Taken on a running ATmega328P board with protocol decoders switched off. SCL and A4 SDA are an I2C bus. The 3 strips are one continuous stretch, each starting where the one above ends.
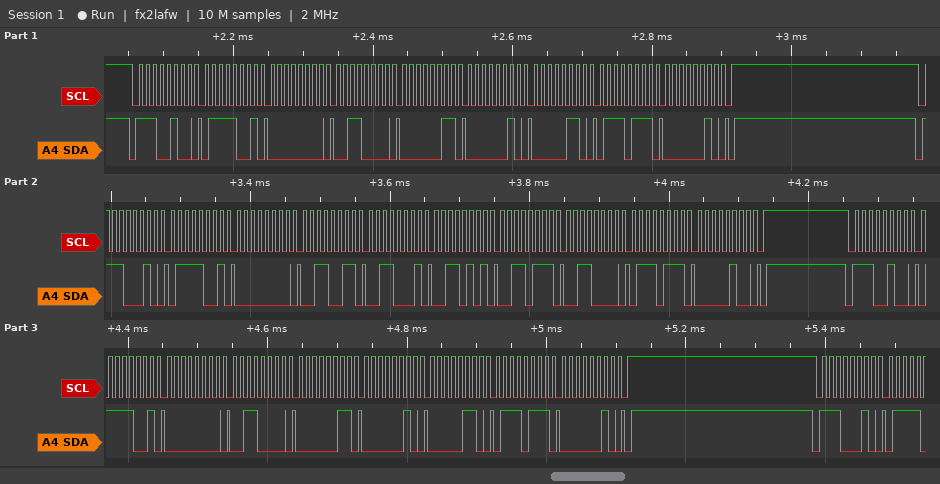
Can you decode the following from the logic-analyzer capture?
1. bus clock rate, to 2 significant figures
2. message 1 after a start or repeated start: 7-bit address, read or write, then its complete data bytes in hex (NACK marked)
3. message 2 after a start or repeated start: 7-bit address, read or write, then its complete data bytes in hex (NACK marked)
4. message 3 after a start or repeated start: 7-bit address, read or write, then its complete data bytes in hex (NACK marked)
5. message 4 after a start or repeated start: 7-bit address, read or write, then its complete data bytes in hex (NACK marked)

100 kHz
0x72 write: 79 00 30 03 02 06 77 02
0x71 write: 79 00 33 31 35 37 30 77 04
0x72 write: 79 00 30 03 02 06 77 02
0x71 write
